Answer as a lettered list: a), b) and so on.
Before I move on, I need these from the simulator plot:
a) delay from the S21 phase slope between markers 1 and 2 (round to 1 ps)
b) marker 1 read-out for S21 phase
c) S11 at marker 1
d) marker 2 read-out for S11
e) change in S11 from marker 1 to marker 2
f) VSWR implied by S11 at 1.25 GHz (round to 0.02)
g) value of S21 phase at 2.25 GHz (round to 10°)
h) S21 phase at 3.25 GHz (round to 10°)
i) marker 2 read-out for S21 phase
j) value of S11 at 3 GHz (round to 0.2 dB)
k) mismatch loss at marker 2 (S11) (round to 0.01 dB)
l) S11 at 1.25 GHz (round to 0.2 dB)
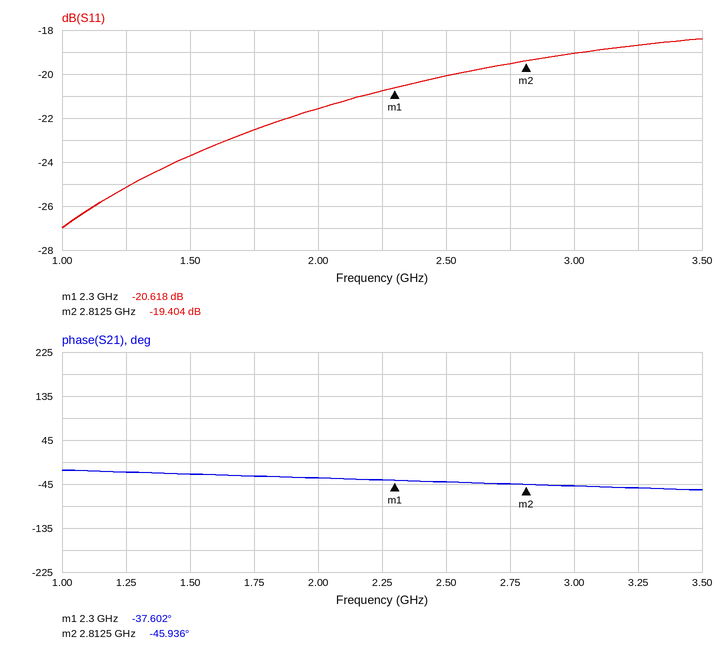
a) 45 ps
b) -37.602°
c) -20.618 dB
d) -19.404 dB
e) 1.214 dB
f) 1.12
g) -40°
h) -50°
i) -45.936°
j) -19.0 dB
k) 0.05 dB
l) -25.2 dB
